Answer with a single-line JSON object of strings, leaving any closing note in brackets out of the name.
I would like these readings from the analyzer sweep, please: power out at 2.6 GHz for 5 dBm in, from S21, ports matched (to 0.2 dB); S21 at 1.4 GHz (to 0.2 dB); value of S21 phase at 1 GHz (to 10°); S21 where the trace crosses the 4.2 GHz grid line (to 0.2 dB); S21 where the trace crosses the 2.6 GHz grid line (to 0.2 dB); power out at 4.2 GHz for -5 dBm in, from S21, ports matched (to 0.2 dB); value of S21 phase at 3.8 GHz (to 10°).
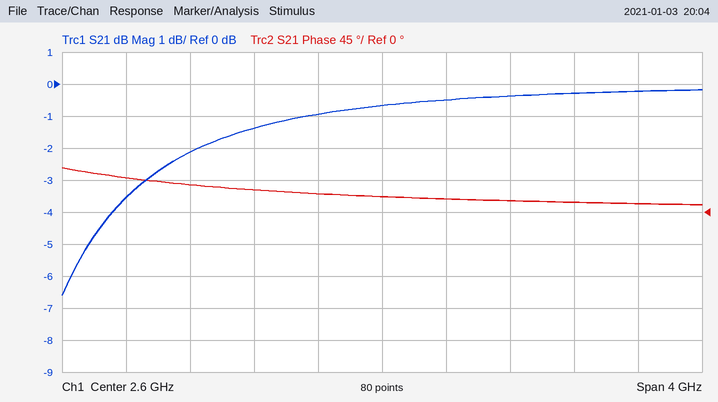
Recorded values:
{"power out at 2.6 GHz for 5 dBm in, from S21, ports matched": "4.4 dBm", "S21 at 1.4 GHz": "-2.2 dB", "value of S21 phase at 1 GHz": "50°", "S21 where the trace crosses the 4.2 GHz grid line": "-0.2 dB", "S21 where the trace crosses the 2.6 GHz grid line": "-0.6 dB", "power out at 4.2 GHz for -5 dBm in, from S21, ports matched": "-5.2 dBm", "value of S21 phase at 3.8 GHz": "10°"}
